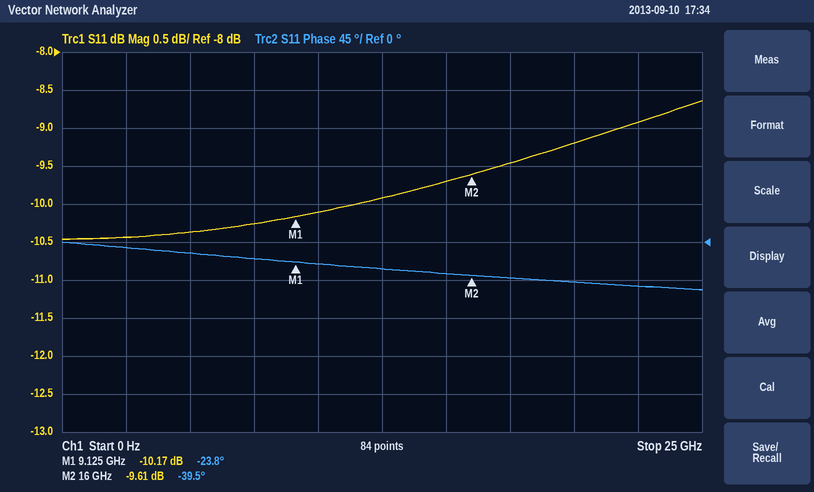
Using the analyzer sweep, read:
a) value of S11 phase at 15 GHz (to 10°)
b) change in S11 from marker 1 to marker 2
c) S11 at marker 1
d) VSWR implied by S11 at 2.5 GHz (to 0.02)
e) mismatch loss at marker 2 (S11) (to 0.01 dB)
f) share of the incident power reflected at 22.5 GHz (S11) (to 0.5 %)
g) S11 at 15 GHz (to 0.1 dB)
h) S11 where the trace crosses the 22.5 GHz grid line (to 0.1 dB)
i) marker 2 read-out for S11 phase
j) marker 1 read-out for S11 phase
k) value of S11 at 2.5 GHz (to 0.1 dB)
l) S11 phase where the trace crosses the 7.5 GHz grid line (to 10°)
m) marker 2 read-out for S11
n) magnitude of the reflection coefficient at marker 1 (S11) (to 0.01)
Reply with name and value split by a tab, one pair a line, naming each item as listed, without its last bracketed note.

value of S11 phase at 15 GHz	-40°
change in S11 from marker 1 to marker 2	0.56 dB
S11 at marker 1	-10.17 dB
VSWR implied by S11 at 2.5 GHz	1.86
mismatch loss at marker 2 (S11)	0.50 dB
share of the incident power reflected at 22.5 GHz (S11)	13.0 %
S11 at 15 GHz	-9.7 dB
S11 where the trace crosses the 22.5 GHz grid line	-8.9 dB
marker 2 read-out for S11 phase	-39.5°
marker 1 read-out for S11 phase	-23.8°
value of S11 at 2.5 GHz	-10.4 dB
S11 phase where the trace crosses the 7.5 GHz grid line	-20°
marker 2 read-out for S11	-9.61 dB
magnitude of the reflection coefficient at marker 1 (S11)	0.31
